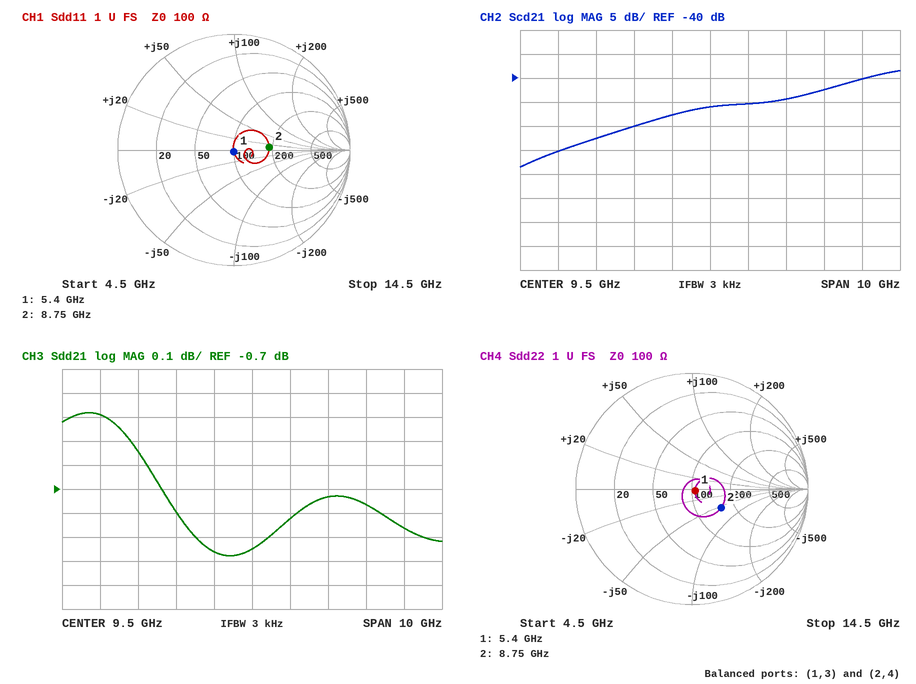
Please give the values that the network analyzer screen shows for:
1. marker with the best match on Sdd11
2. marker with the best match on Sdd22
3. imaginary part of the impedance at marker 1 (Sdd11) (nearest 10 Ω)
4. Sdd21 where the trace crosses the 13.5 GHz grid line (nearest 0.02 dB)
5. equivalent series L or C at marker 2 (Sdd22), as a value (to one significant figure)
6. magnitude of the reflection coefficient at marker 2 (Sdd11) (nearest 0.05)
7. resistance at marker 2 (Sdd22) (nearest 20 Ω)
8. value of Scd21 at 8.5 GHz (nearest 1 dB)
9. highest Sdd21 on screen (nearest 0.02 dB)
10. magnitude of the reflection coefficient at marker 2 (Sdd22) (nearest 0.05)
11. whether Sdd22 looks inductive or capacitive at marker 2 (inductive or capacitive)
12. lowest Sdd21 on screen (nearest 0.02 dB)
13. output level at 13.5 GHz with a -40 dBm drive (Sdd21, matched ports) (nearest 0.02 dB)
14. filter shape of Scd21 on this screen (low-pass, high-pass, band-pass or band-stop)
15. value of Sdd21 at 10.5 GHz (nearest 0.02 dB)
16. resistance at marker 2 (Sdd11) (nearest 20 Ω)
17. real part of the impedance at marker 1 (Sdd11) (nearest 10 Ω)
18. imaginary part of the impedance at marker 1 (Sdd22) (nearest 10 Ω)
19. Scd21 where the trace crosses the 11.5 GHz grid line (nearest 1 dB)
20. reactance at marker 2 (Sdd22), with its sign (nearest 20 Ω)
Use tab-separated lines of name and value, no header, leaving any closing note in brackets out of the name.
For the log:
marker with the best match on Sdd11	marker 1
marker with the best match on Sdd22	marker 1
imaginary part of the impedance at marker 1 (Sdd11)	0 Ω
Sdd21 where the trace crosses the 13.5 GHz grid line	-0.86 dB
equivalent series L or C at marker 2 (Sdd22), as a value	300 fF
magnitude of the reflection coefficient at marker 2 (Sdd11)	0.30
resistance at marker 2 (Sdd22)	160 Ω
value of Scd21 at 8.5 GHz	-48 dB
highest Sdd21 on screen	-0.38 dB
magnitude of the reflection coefficient at marker 2 (Sdd22)	0.30
whether Sdd22 looks inductive or capacitive at marker 2	capacitive
lowest Sdd21 on screen	-0.98 dB
output level at 13.5 GHz with a -40 dBm drive (Sdd21, matched ports)	-40.86 dBm
filter shape of Scd21 on this screen	high-pass
value of Sdd21 at 10.5 GHz	-0.82 dB
resistance at marker 2 (Sdd11)	180 Ω
real part of the impedance at marker 1 (Sdd11)	100 Ω
imaginary part of the impedance at marker 1 (Sdd22)	0 Ω
Scd21 where the trace crosses the 11.5 GHz grid line	-44 dB
reactance at marker 2 (Sdd22), with its sign	-60 Ω
